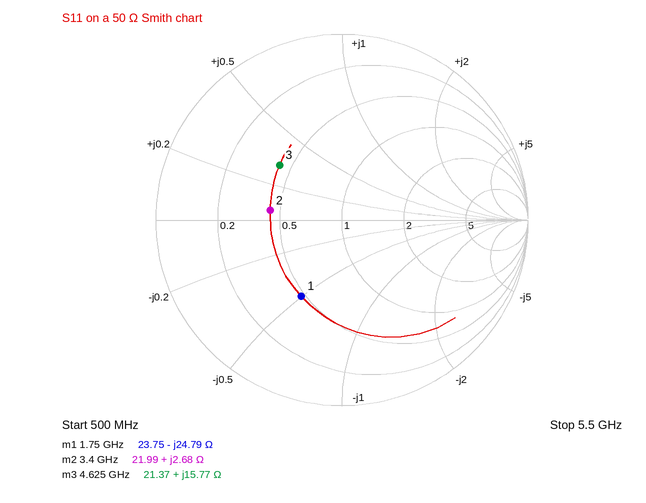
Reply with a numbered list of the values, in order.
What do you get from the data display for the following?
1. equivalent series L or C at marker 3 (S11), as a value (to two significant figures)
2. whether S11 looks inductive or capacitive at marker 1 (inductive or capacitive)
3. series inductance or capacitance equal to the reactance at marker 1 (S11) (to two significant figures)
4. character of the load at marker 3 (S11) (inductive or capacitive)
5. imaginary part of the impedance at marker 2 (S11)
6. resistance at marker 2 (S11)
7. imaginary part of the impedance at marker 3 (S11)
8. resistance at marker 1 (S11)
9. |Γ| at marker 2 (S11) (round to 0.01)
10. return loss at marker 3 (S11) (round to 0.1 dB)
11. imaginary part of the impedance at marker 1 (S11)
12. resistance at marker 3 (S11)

1. 540 pH
2. capacitive
3. 3.7 pF
4. inductive
5. +2.68 Ω
6. 21.99 Ω
7. +15.77 Ω
8. 23.75 Ω
9. 0.39
10. 7.0 dB
11. -24.79 Ω
12. 21.37 Ω
